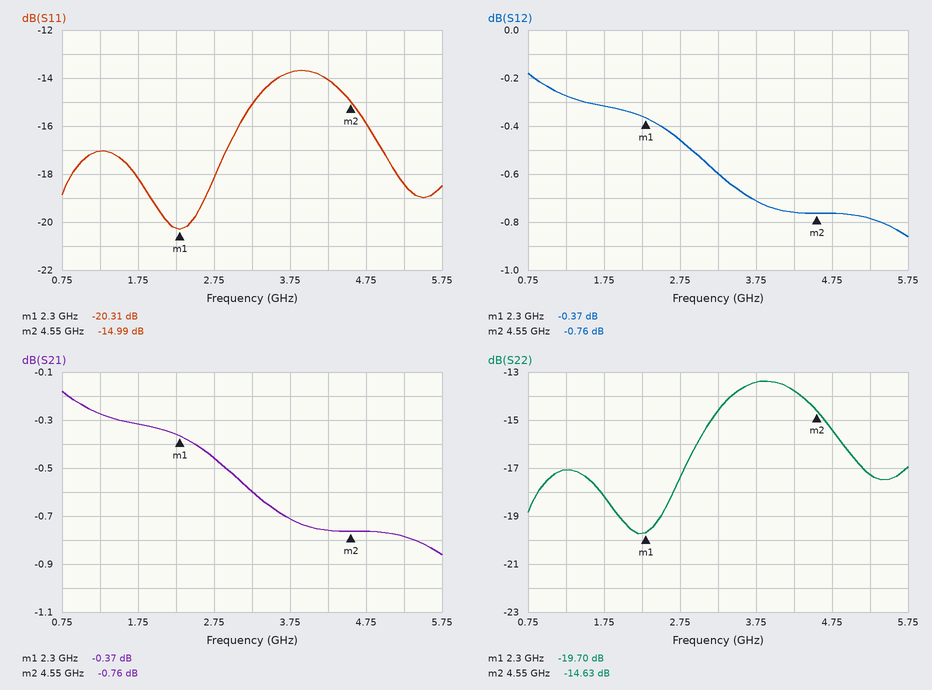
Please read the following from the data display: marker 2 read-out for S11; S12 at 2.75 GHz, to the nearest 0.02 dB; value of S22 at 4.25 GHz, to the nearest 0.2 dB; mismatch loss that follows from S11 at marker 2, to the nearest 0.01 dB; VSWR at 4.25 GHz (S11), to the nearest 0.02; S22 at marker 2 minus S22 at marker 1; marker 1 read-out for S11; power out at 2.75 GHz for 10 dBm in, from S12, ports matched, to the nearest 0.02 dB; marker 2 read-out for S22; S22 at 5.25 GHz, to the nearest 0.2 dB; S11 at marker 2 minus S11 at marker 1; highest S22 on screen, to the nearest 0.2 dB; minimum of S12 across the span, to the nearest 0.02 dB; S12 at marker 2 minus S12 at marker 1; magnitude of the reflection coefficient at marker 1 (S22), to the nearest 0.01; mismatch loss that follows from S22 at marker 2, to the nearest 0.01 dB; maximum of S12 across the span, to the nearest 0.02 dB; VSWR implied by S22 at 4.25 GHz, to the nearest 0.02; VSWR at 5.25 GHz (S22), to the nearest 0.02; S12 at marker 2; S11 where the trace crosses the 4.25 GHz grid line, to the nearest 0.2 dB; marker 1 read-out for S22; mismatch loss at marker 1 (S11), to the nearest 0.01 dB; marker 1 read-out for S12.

-14.99 dB
-0.46 dB
-13.8 dB
0.14 dB
1.50
5.07 dB
-20.31 dB
9.54 dBm
-14.63 dB
-17.2 dB
5.32 dB
-13.4 dB
-0.86 dB
-0.39 dB
0.10
0.15 dB
-0.18 dB
1.52
1.32
-0.76 dB
-14.0 dB
-19.70 dB
0.04 dB
-0.37 dB
